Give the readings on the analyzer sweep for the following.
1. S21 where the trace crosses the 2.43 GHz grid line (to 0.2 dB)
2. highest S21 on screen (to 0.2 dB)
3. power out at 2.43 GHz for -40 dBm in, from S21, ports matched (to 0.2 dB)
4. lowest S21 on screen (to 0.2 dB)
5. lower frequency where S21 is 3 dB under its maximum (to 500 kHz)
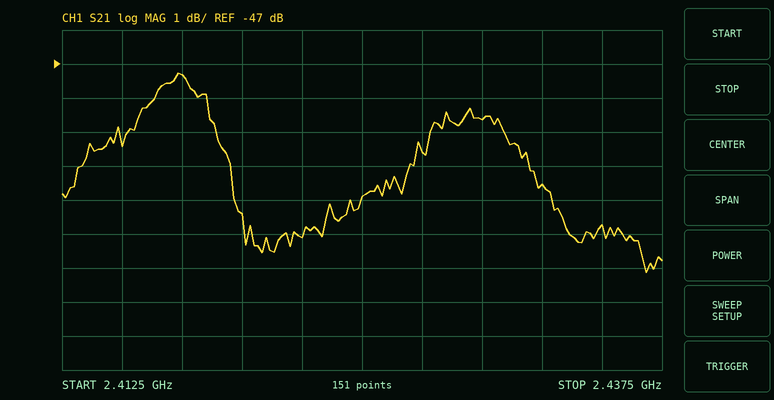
-48.6 dB
-47.2 dB
-88.6 dBm
-53.2 dB
2.4130 GHz
